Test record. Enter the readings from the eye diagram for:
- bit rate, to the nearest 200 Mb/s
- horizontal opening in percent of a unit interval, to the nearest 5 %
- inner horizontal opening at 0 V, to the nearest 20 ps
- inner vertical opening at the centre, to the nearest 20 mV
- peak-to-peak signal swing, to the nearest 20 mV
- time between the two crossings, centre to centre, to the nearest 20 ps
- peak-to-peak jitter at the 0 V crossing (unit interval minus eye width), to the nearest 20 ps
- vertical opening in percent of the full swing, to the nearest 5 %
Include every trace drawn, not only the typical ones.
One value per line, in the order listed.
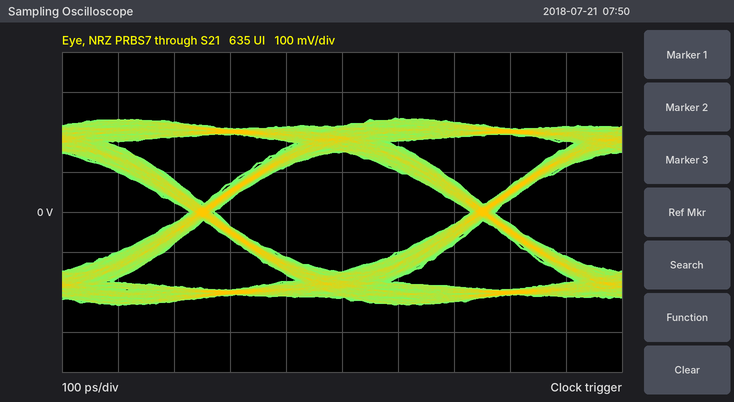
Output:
2.0 Gb/s
90 %
460 ps
300 mV
460 mV
500 ps
40 ps
65 %
